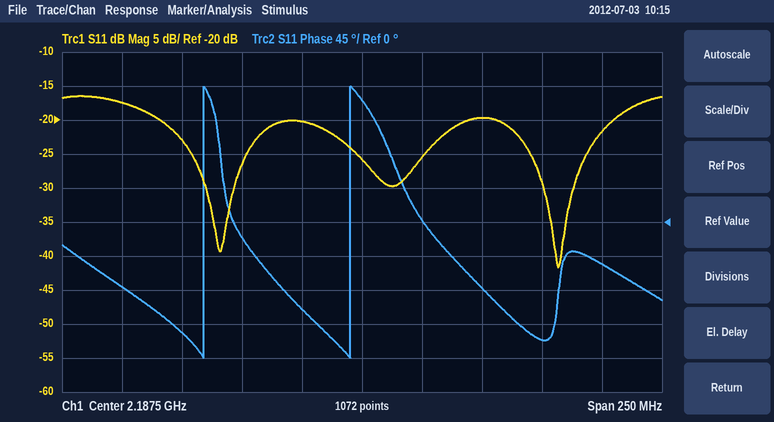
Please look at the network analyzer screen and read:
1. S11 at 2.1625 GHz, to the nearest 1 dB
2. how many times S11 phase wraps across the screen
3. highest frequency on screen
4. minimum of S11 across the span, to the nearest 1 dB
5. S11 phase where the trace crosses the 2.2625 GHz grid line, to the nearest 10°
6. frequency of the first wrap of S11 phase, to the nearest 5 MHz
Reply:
-20 dB
2
2.3125 GHz
-42 dB
-160°
2.120 GHz
